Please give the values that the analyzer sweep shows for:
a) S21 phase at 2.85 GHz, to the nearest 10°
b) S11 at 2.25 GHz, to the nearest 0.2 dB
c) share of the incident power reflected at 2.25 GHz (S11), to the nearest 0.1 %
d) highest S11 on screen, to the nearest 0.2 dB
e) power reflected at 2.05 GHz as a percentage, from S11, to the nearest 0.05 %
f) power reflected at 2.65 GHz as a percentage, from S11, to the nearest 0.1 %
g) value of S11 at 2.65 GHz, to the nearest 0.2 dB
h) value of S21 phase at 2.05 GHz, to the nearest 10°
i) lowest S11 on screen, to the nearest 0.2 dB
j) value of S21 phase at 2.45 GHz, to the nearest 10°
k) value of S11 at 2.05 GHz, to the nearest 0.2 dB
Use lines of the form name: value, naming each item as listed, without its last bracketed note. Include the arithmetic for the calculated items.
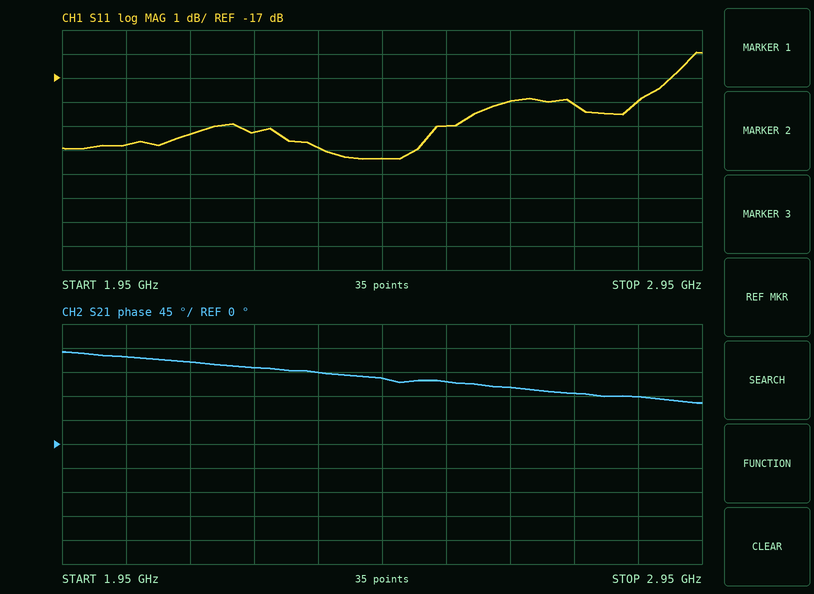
S21 phase at 2.85 GHz, to the nearest 10°: 90°
S11 at 2.25 GHz, to the nearest 0.2 dB: -19.2 dB
share of the incident power reflected at 2.25 GHz (S11), to the nearest 0.1 %: 10^(-19.2/10) ≈ 1.2 %
highest S11 on screen, to the nearest 0.2 dB: -16.0 dB
power reflected at 2.05 GHz as a percentage, from S11, to the nearest 0.05 %: 10^(-19.8/10) ≈ 1.05 %
power reflected at 2.65 GHz as a percentage, from S11, to the nearest 0.1 %: 10^(-18/10) ≈ 1.6 %
value of S11 at 2.65 GHz, to the nearest 0.2 dB: -18.0 dB
value of S21 phase at 2.05 GHz, to the nearest 10°: 160°
lowest S11 on screen, to the nearest 0.2 dB: -20.4 dB
value of S21 phase at 2.45 GHz, to the nearest 10°: 120°
value of S11 at 2.05 GHz, to the nearest 0.2 dB: -19.8 dB
